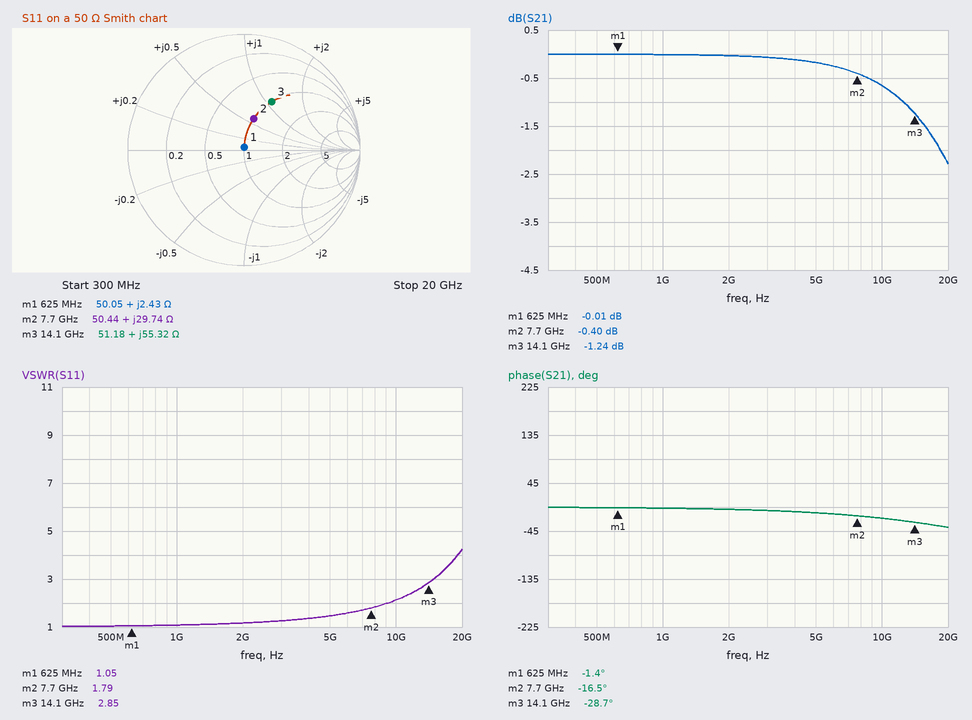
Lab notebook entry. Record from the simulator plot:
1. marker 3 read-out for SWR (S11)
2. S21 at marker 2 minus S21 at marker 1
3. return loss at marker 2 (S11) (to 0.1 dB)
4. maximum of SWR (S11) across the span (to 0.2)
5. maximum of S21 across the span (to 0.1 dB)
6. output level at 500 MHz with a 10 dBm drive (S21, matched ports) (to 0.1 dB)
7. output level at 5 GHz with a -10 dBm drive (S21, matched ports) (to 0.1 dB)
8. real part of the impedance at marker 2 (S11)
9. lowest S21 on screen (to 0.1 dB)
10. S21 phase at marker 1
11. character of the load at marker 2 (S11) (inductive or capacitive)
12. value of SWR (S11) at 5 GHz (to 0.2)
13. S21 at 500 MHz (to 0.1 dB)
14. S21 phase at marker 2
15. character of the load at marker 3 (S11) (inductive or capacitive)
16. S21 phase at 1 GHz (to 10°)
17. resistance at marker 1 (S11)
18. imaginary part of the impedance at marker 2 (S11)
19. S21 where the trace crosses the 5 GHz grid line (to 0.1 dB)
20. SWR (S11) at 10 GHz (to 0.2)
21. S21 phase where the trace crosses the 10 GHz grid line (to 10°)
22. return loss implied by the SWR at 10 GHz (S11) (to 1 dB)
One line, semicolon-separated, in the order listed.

2.85; -0.39 dB; 10.9 dB; 4.2; 0.0 dB; 10.0 dBm; -10.2 dBm; 50.44 Ω; -2.3 dB; -1.4°; inductive; 1.4; 0.0 dB; -16.5°; inductive; 0°; 50.05 Ω; +29.74 Ω; -0.2 dB; 2.2; -20°; 9 dB
